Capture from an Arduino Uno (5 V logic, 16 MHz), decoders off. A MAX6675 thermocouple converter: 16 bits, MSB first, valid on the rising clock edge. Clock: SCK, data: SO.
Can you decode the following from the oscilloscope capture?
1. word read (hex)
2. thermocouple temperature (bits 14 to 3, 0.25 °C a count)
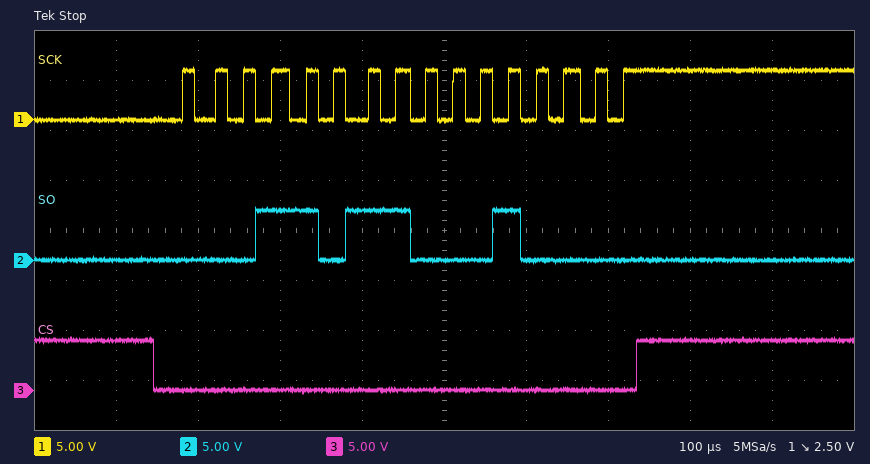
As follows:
0x1B10
216.50 °C
